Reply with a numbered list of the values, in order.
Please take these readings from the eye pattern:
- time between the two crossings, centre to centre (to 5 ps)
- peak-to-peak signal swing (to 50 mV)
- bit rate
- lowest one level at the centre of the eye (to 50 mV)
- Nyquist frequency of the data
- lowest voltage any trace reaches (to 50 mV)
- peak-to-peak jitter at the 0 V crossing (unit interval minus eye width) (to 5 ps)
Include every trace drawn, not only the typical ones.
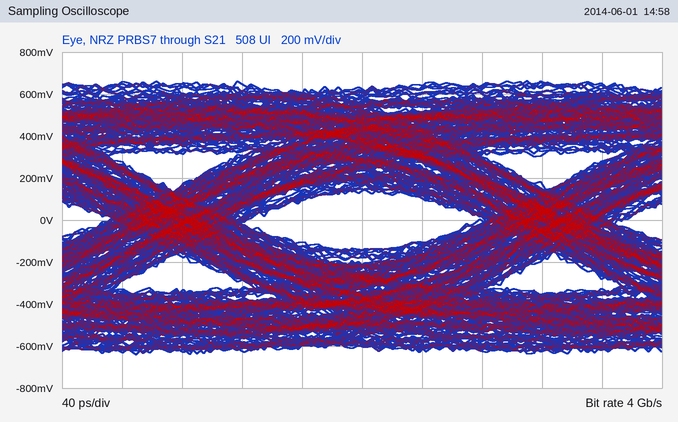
1. 250 ps
2. 1.30 V
3. 4 Gb/s
4. 150 mV
5. 2 GHz
6. -650 mV
7. 95 ps
